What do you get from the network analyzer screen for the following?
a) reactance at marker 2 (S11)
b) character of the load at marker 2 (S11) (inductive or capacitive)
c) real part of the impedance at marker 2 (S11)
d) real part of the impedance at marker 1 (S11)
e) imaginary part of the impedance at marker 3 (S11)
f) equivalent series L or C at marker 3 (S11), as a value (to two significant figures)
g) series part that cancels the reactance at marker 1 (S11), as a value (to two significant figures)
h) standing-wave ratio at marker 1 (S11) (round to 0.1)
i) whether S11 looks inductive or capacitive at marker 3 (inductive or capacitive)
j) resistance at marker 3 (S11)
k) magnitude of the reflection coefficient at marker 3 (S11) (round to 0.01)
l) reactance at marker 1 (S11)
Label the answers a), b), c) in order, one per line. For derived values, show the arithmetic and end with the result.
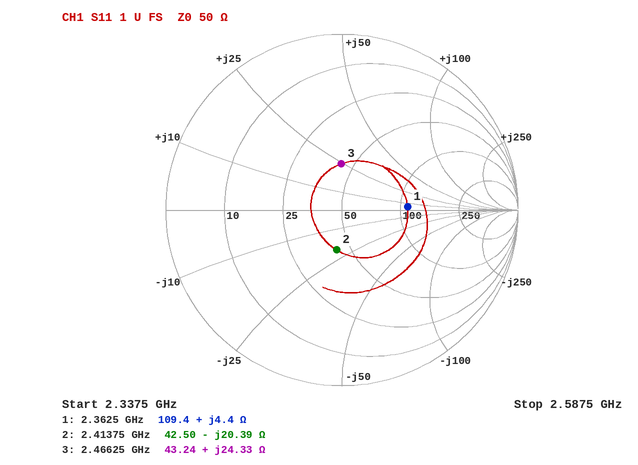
a) -20.39 Ω
b) capacitive
c) 42.50 Ω
d) 109.4 Ω
e) +24.33 Ω
f) L = 24.33 Ω/(2π × 2.46625 GHz) ≈ 1.6 nH
g) C = 1/(2π × 2.3625 GHz × 4.4 Ω) ≈ 15 pF
h) 2.2
i) inductive
j) 43.24 Ω
k) 0.26
l) +4.4 Ω
